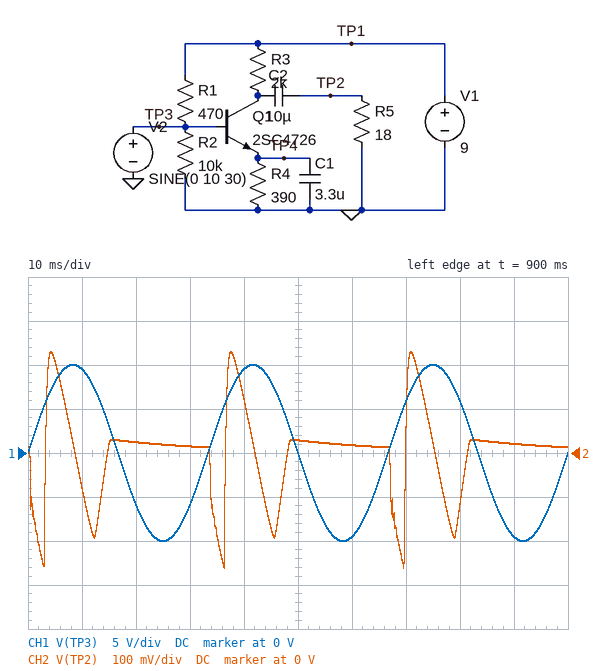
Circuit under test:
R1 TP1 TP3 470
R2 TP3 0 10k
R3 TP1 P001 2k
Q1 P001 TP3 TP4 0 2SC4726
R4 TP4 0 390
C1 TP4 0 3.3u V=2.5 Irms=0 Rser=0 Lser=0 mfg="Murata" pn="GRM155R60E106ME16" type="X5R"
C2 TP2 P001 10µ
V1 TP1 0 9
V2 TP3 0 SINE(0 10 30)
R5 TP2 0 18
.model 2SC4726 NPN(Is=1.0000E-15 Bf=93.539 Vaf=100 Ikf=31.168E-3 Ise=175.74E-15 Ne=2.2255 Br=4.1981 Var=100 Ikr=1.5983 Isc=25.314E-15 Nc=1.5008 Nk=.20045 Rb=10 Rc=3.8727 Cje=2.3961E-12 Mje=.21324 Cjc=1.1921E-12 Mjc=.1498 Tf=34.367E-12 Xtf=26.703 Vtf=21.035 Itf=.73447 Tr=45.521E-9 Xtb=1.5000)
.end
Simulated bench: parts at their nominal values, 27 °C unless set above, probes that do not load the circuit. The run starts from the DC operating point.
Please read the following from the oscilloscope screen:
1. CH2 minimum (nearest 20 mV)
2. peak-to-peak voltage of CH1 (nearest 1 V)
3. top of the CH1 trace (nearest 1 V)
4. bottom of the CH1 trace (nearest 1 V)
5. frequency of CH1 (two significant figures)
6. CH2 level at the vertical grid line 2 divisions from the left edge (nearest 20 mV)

-260 mV
20 V
10 V
-10 V
30 Hz
20 mV
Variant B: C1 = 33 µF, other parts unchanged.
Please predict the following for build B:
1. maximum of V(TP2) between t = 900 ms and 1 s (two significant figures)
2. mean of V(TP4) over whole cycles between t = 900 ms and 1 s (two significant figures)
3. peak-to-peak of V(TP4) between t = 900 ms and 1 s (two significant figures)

250 mV
4.6 V
7.6 V
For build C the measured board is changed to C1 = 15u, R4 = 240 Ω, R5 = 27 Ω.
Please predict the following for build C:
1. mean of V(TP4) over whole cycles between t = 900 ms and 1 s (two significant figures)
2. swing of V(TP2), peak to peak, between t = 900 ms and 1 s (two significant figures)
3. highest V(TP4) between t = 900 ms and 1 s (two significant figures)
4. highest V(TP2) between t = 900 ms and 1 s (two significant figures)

3.0 V
1.3 V
8.8 V
380 mV
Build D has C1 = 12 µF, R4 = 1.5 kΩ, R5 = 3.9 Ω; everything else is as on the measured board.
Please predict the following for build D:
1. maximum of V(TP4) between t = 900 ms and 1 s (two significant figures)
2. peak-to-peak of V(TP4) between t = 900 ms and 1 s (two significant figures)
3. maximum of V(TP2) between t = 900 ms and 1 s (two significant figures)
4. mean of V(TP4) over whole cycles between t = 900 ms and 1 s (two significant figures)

9.1 V
6.9 V
50 mV
5.3 V
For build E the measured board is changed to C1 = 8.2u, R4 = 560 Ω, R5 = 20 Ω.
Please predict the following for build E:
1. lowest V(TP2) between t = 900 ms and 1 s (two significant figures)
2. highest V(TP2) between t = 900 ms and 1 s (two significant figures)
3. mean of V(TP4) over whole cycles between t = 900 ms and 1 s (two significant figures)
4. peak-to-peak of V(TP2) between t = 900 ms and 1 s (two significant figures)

-360 mV
260 mV
3.2 V
630 mV
